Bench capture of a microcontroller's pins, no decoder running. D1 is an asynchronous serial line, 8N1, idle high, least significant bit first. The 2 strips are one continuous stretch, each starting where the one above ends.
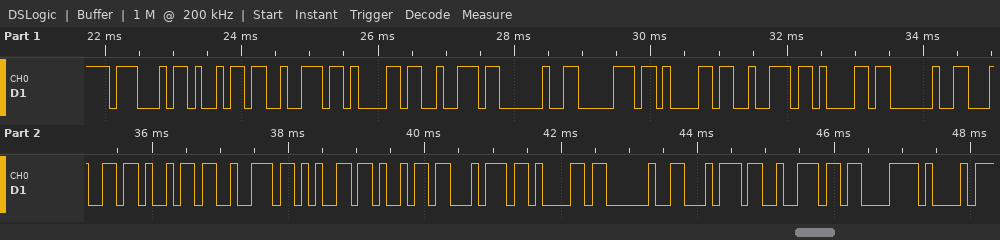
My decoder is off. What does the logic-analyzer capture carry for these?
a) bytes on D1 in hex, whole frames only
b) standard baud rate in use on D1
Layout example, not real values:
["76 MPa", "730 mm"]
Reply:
["47 69 72 61 72 20 70 61 72 61 20 64 69 72 65 69 74 61 20 74 72 C3 A1", "9600 baud"]
